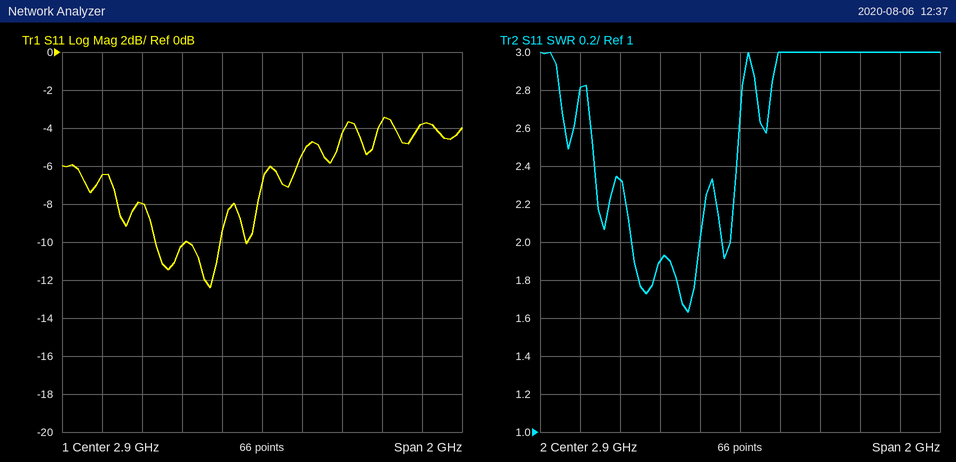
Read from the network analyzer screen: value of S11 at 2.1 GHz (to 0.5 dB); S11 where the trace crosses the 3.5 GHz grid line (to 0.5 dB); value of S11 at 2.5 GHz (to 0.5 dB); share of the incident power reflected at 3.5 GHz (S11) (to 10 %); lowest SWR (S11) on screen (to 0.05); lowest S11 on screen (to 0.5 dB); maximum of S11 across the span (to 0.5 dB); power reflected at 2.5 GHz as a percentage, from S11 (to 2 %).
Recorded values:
-6.5 dB
-3.5 dB
-10.0 dB
40 %
1.65
-12.5 dB
-3.5 dB
10 %
